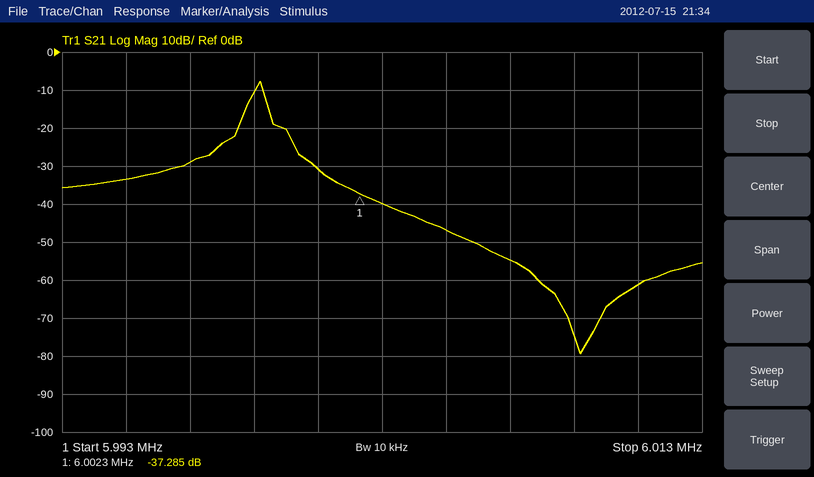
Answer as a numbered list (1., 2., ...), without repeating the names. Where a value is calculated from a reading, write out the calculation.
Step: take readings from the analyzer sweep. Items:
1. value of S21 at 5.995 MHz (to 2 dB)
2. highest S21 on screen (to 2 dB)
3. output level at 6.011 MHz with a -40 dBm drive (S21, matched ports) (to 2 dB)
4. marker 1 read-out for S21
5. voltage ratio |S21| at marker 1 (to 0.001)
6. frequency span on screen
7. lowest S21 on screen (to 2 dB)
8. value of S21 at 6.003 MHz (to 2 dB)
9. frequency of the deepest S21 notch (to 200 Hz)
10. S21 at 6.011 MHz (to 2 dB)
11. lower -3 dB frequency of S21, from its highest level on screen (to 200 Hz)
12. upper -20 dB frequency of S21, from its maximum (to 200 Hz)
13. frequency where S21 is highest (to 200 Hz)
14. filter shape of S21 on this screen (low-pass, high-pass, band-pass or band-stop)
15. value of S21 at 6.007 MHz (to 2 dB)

1. -34 dB
2. -8 dB
3. -40 dBm + (-62 dB) = -102 dBm
4. -37.285 dB
5. 10^(-37.285/20) ≈ 0.014
6. 20 kHz
7. -80 dB
8. -40 dB
9. 6.0092 MHz
10. -62 dB
11. 5.9990 MHz
12. 6.0006 MHz
13. 5.9992 MHz
14. band-pass
15. -54 dB
